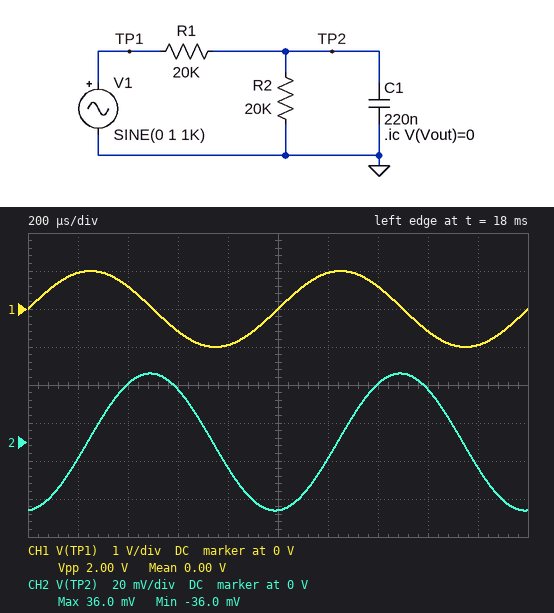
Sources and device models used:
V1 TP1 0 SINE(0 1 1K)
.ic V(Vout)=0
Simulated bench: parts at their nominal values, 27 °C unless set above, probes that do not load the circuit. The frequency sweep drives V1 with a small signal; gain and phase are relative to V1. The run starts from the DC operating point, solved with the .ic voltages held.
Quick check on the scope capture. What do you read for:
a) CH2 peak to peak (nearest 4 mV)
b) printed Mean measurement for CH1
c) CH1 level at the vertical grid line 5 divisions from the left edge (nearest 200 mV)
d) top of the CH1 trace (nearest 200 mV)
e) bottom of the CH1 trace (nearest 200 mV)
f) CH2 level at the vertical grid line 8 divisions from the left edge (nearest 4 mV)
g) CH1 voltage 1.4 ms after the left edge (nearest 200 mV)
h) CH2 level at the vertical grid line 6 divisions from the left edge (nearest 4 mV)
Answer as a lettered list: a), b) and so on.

a) 72 mV
b) 0.00 V
c) 0 V
d) 1.0 V
e) -1.0 V
f) 28 mV
g) 600 mV
h) -8 mV
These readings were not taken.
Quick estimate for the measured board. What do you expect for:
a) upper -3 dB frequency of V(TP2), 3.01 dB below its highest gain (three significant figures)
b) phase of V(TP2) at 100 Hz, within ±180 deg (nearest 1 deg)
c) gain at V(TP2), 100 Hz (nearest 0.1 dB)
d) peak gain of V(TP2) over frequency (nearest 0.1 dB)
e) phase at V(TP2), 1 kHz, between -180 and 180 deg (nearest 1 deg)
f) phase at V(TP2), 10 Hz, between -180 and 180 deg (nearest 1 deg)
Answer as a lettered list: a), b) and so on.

a) 72.3 Hz
b) -54 deg
c) -10.7 dB
d) -6.0 dB
e) -86 deg
f) -8 deg
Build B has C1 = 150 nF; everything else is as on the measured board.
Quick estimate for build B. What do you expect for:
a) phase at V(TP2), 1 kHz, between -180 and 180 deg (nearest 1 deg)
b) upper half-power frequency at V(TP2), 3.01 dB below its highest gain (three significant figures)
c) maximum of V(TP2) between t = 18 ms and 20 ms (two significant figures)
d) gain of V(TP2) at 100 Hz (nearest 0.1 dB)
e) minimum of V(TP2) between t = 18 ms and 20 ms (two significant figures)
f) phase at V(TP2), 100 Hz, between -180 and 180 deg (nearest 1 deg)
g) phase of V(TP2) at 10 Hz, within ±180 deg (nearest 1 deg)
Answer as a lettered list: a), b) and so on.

a) -84 deg
b) 106 Hz
c) 53 mV
d) -8.8 dB
e) -53 mV
f) -43 deg
g) -5 deg
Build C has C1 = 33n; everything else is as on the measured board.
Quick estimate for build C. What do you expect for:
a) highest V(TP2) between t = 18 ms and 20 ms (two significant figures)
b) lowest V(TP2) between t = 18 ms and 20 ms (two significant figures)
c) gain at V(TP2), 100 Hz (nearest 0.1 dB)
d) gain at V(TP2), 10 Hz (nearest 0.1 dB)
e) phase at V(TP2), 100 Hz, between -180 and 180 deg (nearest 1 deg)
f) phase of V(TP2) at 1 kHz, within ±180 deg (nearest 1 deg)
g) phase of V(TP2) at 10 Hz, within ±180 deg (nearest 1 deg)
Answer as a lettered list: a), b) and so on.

a) 220 mV
b) -220 mV
c) -6.2 dB
d) -6.0 dB
e) -12 deg
f) -64 deg
g) -1 deg
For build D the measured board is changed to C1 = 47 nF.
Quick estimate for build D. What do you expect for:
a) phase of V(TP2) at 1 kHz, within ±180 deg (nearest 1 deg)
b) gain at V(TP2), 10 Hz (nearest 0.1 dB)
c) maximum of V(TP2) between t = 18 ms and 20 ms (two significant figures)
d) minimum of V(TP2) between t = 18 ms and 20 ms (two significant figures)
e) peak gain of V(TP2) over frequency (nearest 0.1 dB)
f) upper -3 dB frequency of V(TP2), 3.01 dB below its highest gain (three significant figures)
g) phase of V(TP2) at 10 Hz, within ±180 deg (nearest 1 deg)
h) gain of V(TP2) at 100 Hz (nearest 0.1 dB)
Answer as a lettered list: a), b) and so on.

a) -71 deg
b) -6.0 dB
c) 160 mV
d) -160 mV
e) -6.0 dB
f) 339 Hz
g) -2 deg
h) -6.4 dB
